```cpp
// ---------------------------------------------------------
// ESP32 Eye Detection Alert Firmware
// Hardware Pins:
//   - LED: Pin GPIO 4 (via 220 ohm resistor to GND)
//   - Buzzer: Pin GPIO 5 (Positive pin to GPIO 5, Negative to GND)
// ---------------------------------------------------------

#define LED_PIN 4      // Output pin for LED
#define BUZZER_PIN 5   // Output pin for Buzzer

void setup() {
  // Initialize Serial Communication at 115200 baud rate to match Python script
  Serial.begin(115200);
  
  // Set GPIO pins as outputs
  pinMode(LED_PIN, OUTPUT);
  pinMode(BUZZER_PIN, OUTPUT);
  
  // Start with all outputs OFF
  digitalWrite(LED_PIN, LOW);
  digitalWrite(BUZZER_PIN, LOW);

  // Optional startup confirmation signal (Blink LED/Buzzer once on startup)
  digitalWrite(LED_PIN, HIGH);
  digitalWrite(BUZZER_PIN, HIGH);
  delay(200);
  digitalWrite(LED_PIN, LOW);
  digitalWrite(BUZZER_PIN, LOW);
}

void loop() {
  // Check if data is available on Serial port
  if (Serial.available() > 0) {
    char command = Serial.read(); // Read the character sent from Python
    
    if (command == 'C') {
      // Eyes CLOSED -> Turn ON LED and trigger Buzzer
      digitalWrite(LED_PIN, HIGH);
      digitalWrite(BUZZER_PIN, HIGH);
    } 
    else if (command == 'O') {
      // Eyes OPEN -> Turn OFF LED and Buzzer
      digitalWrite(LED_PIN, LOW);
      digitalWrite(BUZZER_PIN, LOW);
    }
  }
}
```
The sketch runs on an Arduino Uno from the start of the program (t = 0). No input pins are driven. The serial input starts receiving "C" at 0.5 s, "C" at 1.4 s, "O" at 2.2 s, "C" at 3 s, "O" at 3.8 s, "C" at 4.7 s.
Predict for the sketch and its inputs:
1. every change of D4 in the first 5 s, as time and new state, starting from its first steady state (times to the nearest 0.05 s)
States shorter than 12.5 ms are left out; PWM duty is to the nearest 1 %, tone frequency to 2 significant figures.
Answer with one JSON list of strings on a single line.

["0 s high; 0.2 s low; 0.5 s high; 2.2 s low; 3 s high; 3.8 s low; 4.7 s high"]
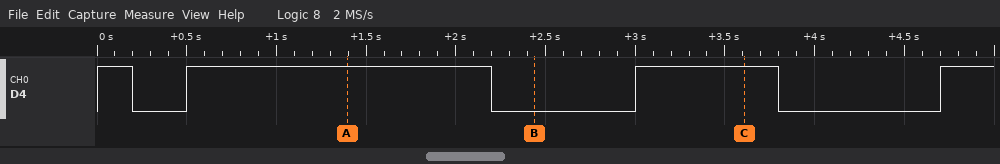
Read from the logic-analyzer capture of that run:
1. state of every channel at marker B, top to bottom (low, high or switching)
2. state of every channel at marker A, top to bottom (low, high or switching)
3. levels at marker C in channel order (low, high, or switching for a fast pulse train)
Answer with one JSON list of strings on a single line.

["D4 low", "D4 high", "D4 high"]
